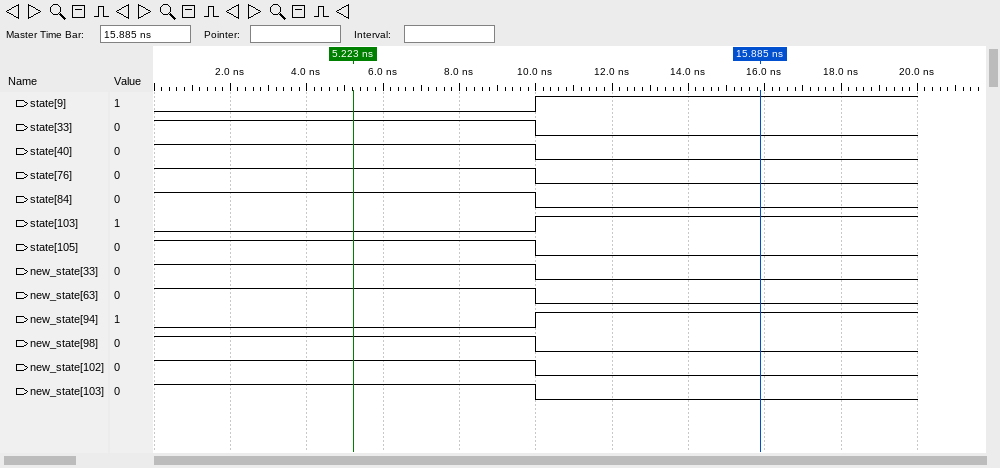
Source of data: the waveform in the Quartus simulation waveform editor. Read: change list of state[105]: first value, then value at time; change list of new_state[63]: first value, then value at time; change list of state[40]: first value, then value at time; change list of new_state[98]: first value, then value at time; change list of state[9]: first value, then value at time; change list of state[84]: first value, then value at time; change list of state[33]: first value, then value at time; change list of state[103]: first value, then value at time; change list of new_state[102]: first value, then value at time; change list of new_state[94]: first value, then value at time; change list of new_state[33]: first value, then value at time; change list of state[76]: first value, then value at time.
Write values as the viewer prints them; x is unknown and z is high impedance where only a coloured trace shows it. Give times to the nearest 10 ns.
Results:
1, 0 at 10 ns
1, 0 at 10 ns
1, 0 at 10 ns
1, 0 at 10 ns
0, 1 at 10 ns
1, 0 at 10 ns
1, 0 at 10 ns
0, 1 at 10 ns
1, 0 at 10 ns
0, 1 at 10 ns
1, 0 at 10 ns
1, 0 at 10 ns
